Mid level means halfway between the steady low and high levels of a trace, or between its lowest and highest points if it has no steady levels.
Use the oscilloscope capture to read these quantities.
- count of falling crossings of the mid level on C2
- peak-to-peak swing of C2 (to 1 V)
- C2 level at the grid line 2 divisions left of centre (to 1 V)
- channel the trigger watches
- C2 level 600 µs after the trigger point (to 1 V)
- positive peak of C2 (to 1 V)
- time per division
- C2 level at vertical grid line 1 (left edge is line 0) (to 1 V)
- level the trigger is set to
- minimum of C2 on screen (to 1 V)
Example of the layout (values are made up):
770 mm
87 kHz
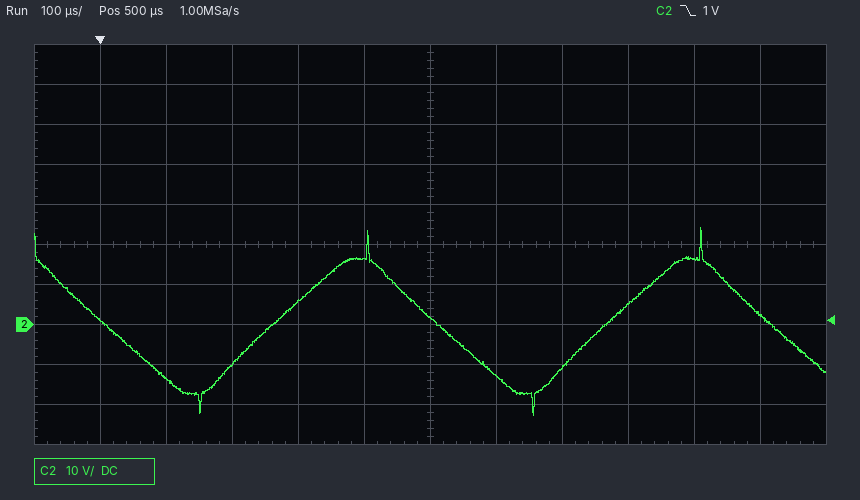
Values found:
3
47 V
6 V
C2
-13 V
24 V
100 µs
1 V
1 V
-23 V
